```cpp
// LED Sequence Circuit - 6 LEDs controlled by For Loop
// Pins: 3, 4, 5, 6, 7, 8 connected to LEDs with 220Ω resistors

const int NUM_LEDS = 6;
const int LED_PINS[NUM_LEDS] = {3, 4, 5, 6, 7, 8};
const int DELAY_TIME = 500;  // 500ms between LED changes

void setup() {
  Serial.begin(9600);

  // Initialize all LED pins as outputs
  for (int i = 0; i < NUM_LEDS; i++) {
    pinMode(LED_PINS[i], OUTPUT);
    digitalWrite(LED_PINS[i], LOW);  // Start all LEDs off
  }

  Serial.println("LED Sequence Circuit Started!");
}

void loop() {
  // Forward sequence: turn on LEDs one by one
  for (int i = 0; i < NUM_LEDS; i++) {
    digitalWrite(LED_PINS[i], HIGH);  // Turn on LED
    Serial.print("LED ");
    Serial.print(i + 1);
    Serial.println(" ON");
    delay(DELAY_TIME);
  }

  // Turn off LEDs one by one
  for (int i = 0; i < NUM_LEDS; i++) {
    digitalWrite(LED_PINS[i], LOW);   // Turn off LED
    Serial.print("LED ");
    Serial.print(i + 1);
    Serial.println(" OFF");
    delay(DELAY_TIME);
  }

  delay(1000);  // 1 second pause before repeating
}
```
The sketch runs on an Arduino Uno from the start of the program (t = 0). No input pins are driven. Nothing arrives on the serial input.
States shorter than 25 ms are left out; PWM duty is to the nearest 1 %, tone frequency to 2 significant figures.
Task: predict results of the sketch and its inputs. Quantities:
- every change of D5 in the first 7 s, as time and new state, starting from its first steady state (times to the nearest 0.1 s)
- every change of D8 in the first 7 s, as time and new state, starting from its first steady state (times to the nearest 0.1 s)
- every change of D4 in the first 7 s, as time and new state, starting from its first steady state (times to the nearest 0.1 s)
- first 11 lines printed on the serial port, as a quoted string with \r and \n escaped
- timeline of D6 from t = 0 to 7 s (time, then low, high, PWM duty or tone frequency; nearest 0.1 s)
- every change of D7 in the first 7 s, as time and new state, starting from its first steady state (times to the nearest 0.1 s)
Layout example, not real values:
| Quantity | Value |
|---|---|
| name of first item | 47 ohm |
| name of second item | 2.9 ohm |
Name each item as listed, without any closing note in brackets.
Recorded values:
| Quantity | Value |
|---|---|
| every change of D5 in the first 7 s, as time and new state, starting from its first steady state | 0 s low; 1 s high; 4 s low |
| every change of D8 in the first 7 s, as time and new state, starting from its first steady state | 0 s low; 2.5 s high; 5.5 s low |
| every change of D4 in the first 7 s, as time and new state, starting from its first steady state | 0 s low; 0.5 s high; 3.5 s low |
| first 11 lines printed on the serial port, as a quoted string with \r and \n escaped | "LED Sequence Circuit Started!\r\nLED 1 ON\r\nLED 2 ON\r\nLED 3 ON\r\nLED 4 ON\r\nLED 5 ON\r\nLED 6 ON\r\nLED 1 OFF\r\nLED 2 OFF\r\nLED 3 OFF\r\nLED 4 OFF\r\n" |
| timeline of D6 from t = 0 to 7 s | 0 s low; 1.5 s high; 4.5 s low |
| every change of D7 in the first 7 s, as time and new state, starting from its first steady state | 0 s low; 2 s high; 5 s low |
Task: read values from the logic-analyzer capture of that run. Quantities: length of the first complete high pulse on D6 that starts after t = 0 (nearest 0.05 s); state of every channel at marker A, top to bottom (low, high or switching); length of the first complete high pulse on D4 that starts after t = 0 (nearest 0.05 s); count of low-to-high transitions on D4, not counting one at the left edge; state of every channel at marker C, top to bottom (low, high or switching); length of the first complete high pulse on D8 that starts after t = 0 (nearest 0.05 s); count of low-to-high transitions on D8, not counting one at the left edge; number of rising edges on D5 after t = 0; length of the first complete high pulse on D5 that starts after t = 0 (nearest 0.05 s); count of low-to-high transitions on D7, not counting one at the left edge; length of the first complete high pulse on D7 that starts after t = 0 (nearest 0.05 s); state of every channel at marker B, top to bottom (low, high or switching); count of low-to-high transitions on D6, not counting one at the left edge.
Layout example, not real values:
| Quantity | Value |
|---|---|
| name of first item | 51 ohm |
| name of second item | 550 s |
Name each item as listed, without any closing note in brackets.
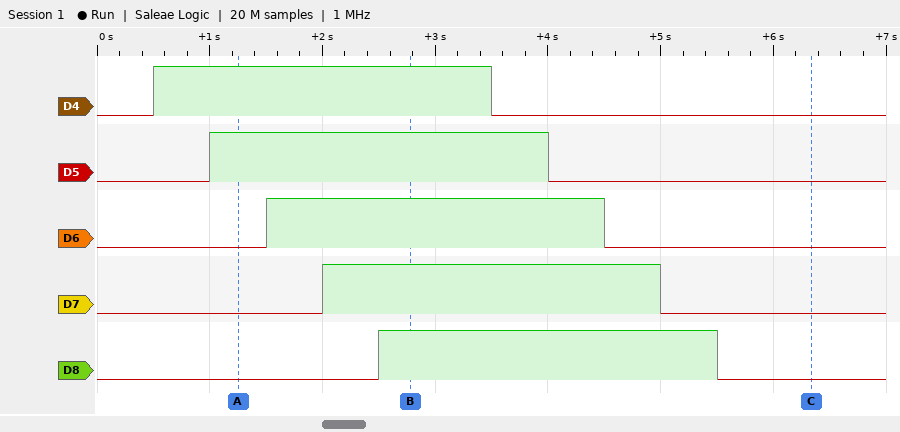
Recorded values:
| Quantity | Value |
|---|---|
| length of the first complete high pulse on D6 that starts after t = 0 | 3.00 s |
| state of every channel at marker A, top to bottom | D4 high, D5 high, D6 low, D7 low, D8 low |
| length of the first complete high pulse on D4 that starts after t = 0 | 3.00 s |
| count of low-to-high transitions on D4, not counting one at the left edge | 1 |
| state of every channel at marker C, top to bottom | D4 low, D5 low, D6 low, D7 low, D8 low |
| length of the first complete high pulse on D8 that starts after t = 0 | 3.00 s |
| count of low-to-high transitions on D8, not counting one at the left edge | 1 |
| number of rising edges on D5 after t = 0 | 1 |
| length of the first complete high pulse on D5 that starts after t = 0 | 3.00 s |
| count of low-to-high transitions on D7, not counting one at the left edge | 1 |
| length of the first complete high pulse on D7 that starts after t = 0 | 3.00 s |
| state of every channel at marker B, top to bottom | D4 high, D5 high, D6 high, D7 high, D8 high |
| count of low-to-high transitions on D6, not counting one at the left edge | 1 |
